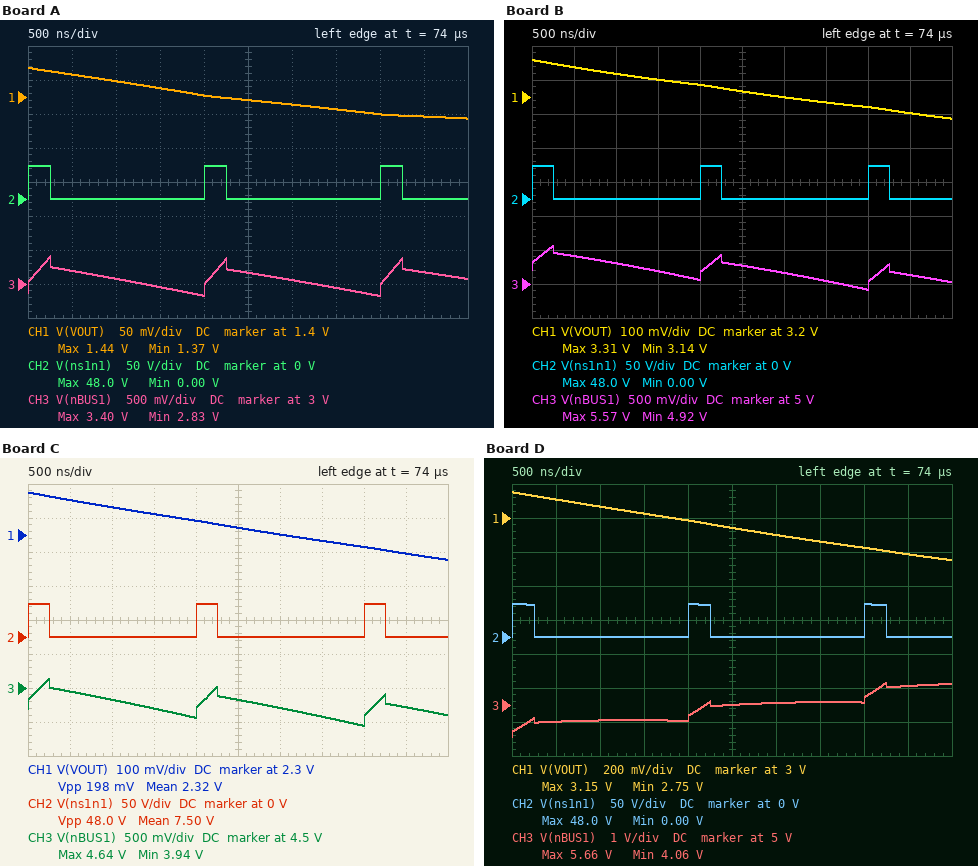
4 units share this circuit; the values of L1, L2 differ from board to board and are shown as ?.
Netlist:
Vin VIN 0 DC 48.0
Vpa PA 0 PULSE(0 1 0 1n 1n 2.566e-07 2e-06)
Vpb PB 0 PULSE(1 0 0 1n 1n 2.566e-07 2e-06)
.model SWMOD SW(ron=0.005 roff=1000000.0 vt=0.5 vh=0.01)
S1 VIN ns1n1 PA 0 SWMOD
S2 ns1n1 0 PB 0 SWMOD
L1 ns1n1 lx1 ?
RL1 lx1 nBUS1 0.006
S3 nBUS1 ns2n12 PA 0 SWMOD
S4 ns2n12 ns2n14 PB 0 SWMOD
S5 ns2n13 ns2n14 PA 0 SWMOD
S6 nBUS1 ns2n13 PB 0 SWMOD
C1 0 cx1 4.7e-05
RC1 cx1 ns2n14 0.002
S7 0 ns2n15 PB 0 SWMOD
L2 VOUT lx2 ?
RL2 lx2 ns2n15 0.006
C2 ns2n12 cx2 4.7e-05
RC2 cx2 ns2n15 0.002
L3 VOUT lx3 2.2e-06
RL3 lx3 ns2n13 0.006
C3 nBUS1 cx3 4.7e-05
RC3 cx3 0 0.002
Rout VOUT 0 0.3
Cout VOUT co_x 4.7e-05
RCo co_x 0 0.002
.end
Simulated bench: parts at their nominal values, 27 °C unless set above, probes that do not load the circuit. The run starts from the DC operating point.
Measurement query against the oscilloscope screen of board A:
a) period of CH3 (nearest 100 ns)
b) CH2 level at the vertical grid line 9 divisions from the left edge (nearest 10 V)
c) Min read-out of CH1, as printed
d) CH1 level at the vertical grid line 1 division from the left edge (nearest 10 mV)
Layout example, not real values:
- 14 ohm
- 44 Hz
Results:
- 2.0 µs
- 0 V
- 1.37 V
- 1.43 V
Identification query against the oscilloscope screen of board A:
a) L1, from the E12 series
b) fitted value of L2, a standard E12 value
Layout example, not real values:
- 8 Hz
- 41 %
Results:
- 5.6 µH
- 1.5 µH
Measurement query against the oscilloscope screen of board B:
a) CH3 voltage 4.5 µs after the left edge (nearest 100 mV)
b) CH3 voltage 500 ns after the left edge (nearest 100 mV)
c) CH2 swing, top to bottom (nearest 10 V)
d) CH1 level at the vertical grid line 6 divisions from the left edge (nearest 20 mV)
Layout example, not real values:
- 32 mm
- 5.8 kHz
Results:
- 5.1 V
- 5.4 V
- 50 V
- 3.20 V
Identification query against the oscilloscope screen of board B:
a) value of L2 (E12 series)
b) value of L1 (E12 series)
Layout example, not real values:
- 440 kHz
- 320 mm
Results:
- 6.8 µH
- 3.9 µH
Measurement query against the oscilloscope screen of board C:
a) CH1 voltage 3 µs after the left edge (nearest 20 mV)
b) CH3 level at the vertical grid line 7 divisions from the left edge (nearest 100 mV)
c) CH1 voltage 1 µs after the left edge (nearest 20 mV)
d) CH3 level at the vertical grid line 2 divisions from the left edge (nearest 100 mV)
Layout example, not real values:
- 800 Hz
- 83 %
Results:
- 2.30 V
- 4.1 V
- 2.38 V
- 4.3 V
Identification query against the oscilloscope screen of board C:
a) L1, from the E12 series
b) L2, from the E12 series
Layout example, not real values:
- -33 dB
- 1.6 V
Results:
- 5.6 µH
- 3.3 µH
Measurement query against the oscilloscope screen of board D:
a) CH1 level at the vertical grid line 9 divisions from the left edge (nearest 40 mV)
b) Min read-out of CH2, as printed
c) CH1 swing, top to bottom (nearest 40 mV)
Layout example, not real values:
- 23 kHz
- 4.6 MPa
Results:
- 2.80 V
- 0.00 V
- 400 mV
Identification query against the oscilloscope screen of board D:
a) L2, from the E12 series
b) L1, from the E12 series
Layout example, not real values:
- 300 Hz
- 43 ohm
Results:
- 4.7 µH
- 1 µH
